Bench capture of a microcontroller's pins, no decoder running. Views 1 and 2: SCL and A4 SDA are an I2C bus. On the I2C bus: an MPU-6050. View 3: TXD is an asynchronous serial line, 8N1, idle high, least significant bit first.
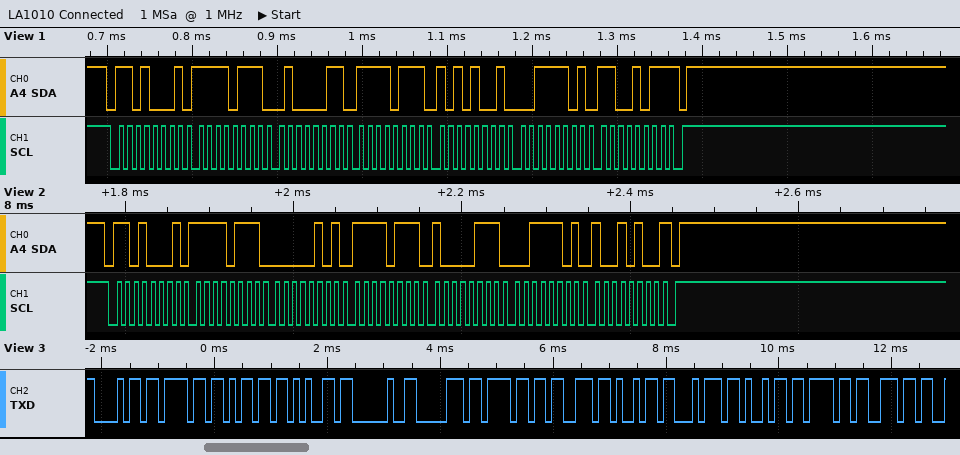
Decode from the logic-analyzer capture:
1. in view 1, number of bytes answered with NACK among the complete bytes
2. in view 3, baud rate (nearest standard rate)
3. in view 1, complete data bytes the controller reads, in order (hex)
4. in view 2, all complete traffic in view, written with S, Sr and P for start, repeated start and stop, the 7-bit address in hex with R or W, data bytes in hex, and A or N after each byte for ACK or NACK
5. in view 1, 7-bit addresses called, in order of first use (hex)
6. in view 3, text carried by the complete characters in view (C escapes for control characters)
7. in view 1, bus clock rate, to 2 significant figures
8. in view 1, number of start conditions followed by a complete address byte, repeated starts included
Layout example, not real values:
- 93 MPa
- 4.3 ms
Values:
- 1
- 9600 baud
- F7 43 F7 A9 3D CB
- S 68R A F7 A 05 A F7 A 87 A 3D A 94 N P
- 0x68
- "home position"
- 100 kHz
- 1
